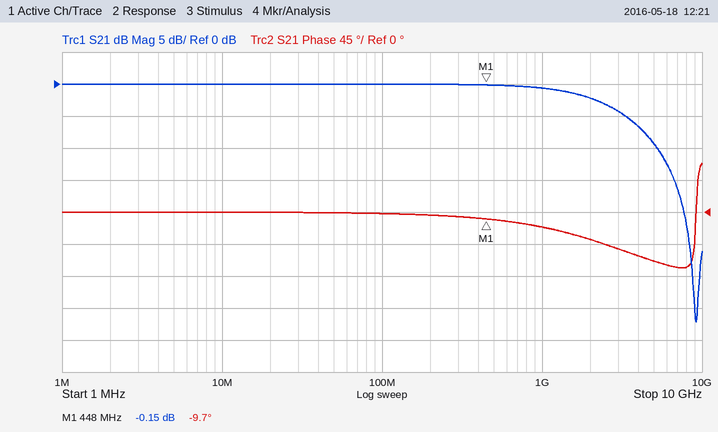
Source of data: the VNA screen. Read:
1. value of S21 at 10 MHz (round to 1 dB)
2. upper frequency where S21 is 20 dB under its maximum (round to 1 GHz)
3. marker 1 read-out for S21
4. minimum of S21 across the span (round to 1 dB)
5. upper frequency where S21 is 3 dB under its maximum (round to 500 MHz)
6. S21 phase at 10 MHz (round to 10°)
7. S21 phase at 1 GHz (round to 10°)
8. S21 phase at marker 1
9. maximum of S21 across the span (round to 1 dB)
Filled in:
0 dB
8 GHz
-0.15 dB
-37 dB
2.5 GHz
0°
-20°
-9.7°
0 dB
